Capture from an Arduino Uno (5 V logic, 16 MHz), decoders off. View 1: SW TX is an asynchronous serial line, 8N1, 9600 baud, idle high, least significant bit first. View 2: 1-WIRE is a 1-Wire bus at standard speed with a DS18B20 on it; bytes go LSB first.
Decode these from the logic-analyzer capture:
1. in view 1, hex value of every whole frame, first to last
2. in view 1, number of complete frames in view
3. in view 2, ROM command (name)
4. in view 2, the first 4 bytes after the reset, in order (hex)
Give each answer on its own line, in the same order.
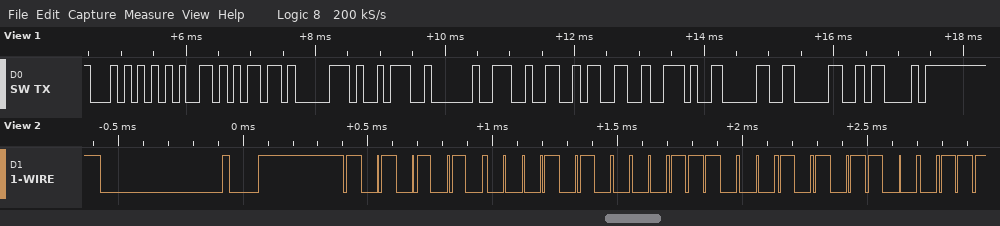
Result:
54 65 6D 70 3A 20 32 33 2E 30 30 43
12
Match ROM
55 28 1C 35
